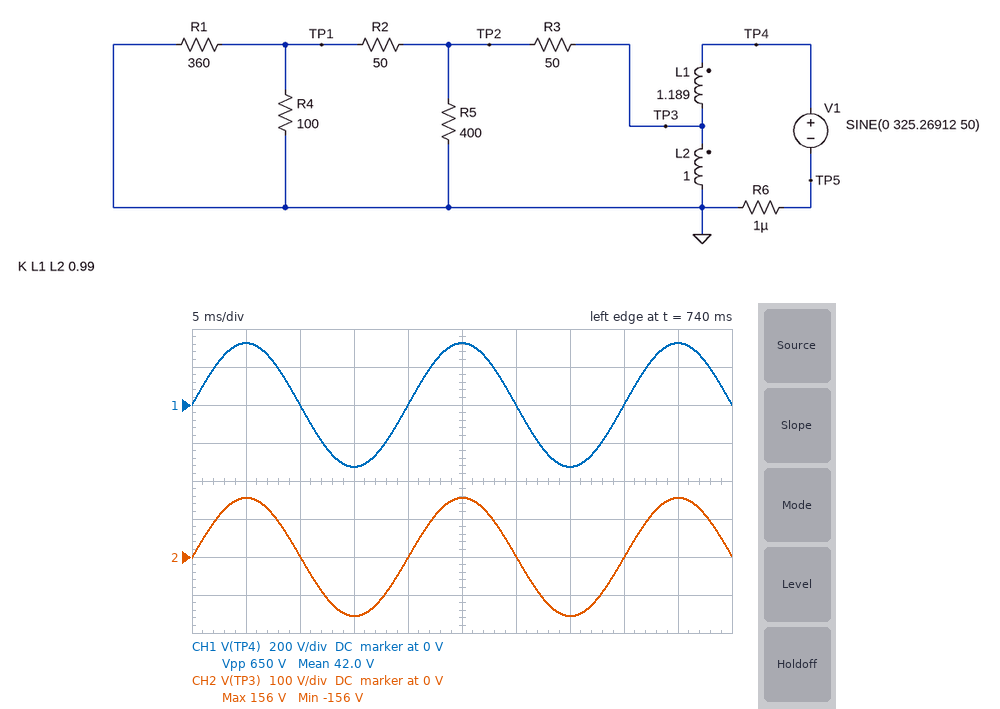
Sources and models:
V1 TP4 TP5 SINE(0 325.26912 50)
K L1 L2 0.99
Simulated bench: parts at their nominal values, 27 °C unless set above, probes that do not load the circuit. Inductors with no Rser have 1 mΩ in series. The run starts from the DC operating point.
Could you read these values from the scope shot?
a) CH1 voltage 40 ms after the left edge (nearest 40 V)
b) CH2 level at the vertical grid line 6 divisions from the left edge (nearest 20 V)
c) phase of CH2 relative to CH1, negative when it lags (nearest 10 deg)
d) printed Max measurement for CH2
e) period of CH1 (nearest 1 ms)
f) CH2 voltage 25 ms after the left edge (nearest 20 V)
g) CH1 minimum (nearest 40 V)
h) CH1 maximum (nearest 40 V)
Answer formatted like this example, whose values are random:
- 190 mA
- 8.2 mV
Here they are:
- 0 V
- 0 V
- 0 deg
- 156 V
- 20 ms
- 160 V
- -320 V
- 320 V
